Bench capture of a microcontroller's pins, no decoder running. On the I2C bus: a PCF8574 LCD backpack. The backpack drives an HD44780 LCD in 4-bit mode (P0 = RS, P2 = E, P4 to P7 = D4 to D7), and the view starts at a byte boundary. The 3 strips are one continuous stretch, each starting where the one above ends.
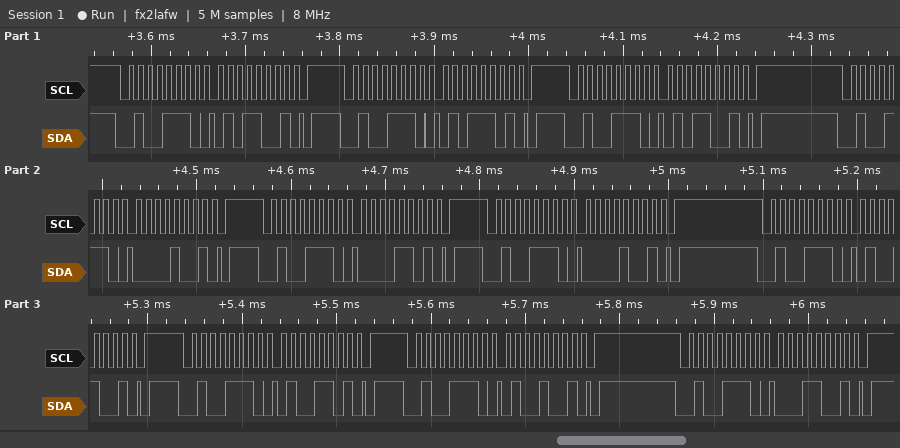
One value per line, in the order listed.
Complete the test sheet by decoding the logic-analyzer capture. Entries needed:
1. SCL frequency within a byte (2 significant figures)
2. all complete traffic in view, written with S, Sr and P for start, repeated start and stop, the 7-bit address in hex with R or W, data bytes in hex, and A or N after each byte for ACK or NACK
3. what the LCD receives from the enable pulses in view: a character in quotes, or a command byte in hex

100 kHz
S 27W A 59 A P S 27W A 5D A P S 27W A 59 A P S 27W A 09 A P S 27W A 0D A P S 27W A 09 A P S 27W A 49 A P S 27W A 4D A P S 27W A 49 A P S 27W A 19 A P
'P'
